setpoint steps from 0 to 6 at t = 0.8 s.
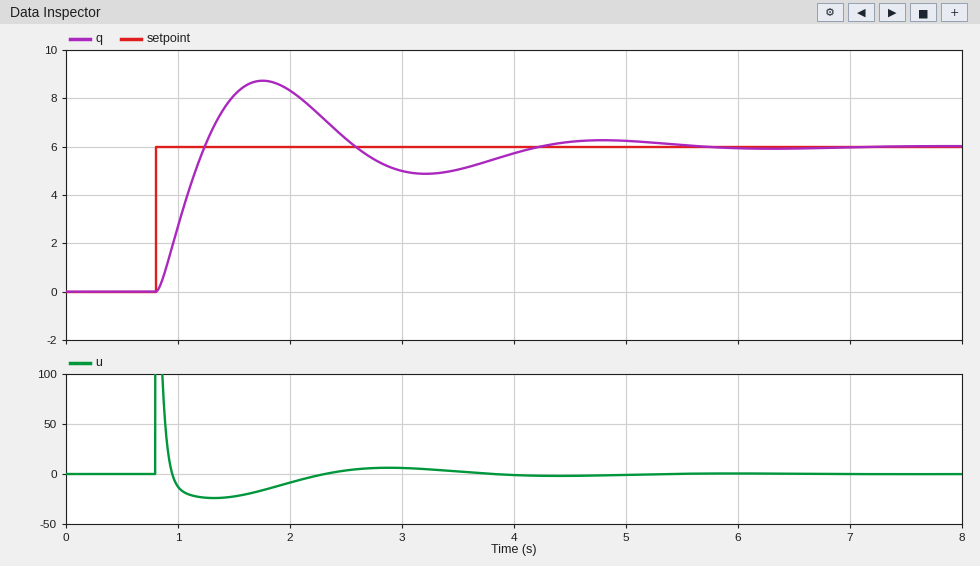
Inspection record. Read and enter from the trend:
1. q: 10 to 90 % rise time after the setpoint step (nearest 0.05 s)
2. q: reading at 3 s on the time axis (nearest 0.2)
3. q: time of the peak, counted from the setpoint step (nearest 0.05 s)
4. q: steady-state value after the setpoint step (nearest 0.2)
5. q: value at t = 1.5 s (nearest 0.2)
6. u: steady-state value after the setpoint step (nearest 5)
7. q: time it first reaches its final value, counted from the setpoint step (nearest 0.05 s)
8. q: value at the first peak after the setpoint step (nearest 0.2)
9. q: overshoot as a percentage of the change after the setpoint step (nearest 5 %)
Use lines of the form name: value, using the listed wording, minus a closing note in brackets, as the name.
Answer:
q: 10 to 90 % rise time after the setpoint step: 0.30 s
q: reading at 3 s on the time axis: 5.0
q: time of the peak, counted from the setpoint step: 0.95 s
q: steady-state value after the setpoint step: 6.0
q: value at t = 1.5 s: 8.2
u: steady-state value after the setpoint step: 0
q: time it first reaches its final value, counted from the setpoint step: 0.45 s
q: value at the first peak after the setpoint step: 8.8
q: overshoot as a percentage of the change after the setpoint step: 45 %
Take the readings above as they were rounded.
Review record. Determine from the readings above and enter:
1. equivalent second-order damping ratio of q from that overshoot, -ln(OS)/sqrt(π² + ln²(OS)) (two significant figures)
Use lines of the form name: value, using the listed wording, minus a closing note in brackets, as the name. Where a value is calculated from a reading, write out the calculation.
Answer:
equivalent second-order damping ratio of q from that overshoot, -ln(OS)/sqrt(π² + ln²(OS)): ln(0.45) = -0.799; 0.799 / sqrt(9.870 + 0.638) = 0.25
